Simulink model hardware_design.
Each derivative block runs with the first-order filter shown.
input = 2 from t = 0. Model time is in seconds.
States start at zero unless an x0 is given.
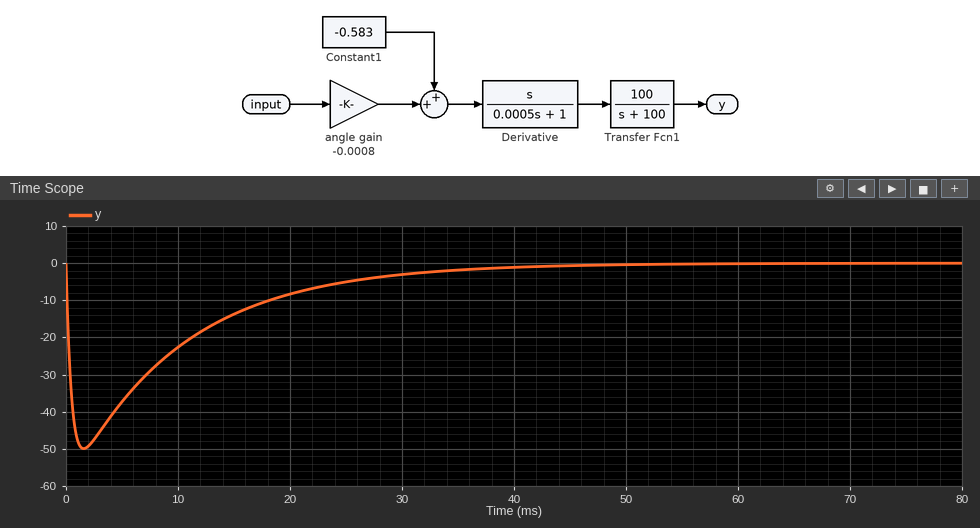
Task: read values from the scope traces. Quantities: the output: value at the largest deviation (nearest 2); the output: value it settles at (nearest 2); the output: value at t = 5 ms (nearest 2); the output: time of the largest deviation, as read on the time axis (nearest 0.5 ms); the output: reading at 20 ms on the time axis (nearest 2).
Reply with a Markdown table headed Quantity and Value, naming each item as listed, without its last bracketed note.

| Quantity | Value |
|---|---|
| the output: value at the largest deviation | -50 |
| the output: value it settles at | 0 |
| the output: value at t = 5 ms | -38 |
| the output: time of the largest deviation, as read on the time axis | 1.5 ms |
| the output: reading at 20 ms on the time axis | -8 |
